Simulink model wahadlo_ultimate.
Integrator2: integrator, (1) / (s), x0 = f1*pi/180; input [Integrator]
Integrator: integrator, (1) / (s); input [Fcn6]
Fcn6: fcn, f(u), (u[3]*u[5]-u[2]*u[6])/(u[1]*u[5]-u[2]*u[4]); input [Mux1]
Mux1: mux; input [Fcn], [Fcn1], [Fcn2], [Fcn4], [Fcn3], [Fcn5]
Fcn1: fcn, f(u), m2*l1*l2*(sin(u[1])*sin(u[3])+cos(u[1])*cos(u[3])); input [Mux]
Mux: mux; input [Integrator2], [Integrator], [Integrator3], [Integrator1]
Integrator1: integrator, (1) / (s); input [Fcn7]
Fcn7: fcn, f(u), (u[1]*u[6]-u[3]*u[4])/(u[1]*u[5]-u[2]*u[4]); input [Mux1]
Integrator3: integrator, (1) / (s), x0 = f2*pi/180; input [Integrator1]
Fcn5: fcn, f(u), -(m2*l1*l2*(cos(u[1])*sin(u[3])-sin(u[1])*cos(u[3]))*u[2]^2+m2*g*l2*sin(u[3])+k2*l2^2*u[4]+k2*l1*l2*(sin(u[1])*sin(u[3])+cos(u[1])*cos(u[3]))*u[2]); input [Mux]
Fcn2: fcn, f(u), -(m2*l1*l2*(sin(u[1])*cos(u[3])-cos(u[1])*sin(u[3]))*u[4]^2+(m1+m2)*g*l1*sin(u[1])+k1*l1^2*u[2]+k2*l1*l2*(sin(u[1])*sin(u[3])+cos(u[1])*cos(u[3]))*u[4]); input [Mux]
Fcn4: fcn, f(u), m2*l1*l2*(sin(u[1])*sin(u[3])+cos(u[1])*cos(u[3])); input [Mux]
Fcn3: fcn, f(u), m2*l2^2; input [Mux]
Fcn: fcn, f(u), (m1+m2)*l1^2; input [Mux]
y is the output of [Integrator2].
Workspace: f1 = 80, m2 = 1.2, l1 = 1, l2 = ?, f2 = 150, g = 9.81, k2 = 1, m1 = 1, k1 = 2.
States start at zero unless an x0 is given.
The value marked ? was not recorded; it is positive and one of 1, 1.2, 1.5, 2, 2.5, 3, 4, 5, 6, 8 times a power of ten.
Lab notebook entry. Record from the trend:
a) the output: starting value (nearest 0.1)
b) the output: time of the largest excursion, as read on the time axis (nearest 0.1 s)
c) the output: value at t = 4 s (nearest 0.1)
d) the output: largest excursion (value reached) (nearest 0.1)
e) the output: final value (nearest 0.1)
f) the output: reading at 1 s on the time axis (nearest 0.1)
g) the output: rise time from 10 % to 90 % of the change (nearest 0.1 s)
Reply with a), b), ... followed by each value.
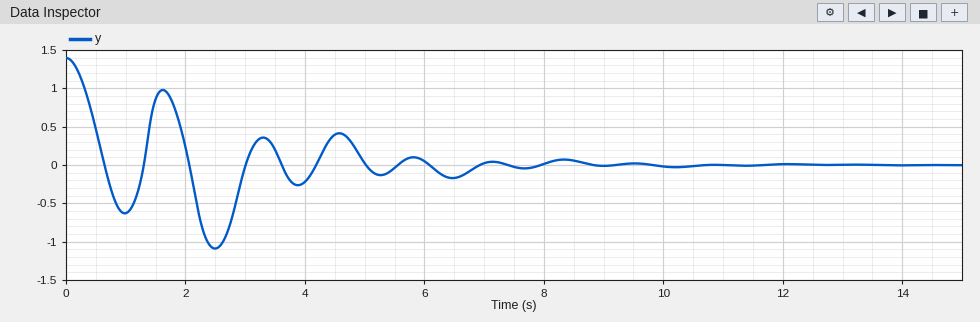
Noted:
a) 1.4
b) 2.5 s
c) -0.2
d) -1.1
e) 0.0
f) -0.6
g) 0.4 s
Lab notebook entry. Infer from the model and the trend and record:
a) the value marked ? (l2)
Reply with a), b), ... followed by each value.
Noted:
a) 3
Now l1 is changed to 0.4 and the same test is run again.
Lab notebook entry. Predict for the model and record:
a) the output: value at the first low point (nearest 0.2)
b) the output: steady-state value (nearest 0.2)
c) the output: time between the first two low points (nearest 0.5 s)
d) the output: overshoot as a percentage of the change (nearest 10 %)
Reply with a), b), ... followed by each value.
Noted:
a) -1.8
b) 0.0
c) 1.5 s
d) 120 %
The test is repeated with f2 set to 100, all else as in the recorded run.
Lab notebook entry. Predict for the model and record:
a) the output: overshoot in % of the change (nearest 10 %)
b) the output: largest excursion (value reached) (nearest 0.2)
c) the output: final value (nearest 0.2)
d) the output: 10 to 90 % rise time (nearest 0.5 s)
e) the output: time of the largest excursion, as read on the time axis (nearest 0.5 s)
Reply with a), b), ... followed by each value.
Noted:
a) 50 %
b) -0.8
c) 0.0
d) 1.5 s
e) 2.0 s
